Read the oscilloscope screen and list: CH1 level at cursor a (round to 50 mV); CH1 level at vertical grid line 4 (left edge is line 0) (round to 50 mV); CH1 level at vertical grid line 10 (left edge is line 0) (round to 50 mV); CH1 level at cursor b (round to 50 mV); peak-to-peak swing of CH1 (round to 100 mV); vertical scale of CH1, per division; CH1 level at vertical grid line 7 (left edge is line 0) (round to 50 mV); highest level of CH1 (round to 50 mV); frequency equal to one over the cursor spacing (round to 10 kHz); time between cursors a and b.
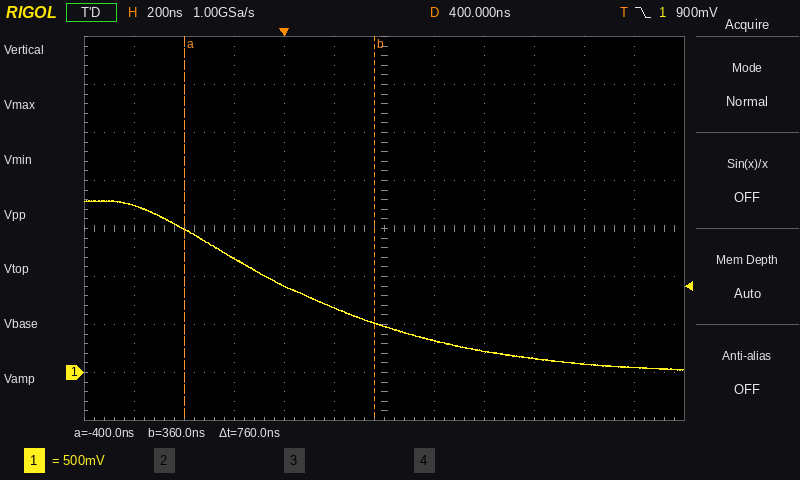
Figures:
1.50 V
900 mV
100 mV
500 mV
1.80 V
500 mV
350 mV
1.80 V
1.32 MHz
760 ns
